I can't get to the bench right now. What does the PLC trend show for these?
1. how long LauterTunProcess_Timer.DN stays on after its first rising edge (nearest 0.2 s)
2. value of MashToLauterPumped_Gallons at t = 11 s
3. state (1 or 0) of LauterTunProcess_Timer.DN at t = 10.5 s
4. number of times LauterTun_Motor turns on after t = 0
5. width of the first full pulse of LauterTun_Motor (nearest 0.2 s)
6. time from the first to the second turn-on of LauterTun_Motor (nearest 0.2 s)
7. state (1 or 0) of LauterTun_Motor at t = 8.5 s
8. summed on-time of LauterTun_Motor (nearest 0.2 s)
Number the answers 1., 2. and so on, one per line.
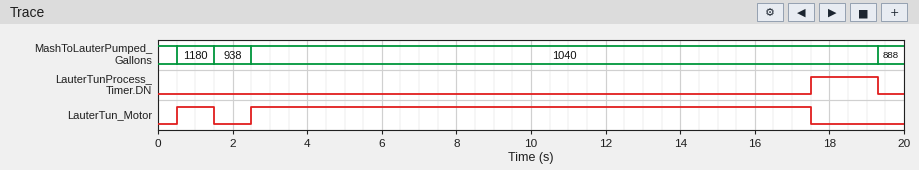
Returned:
1. 1.8 s
2. 1040
3. 0
4. 2
5. 1.0 s
6. 2.0 s
7. 1
8. 16.0 s
